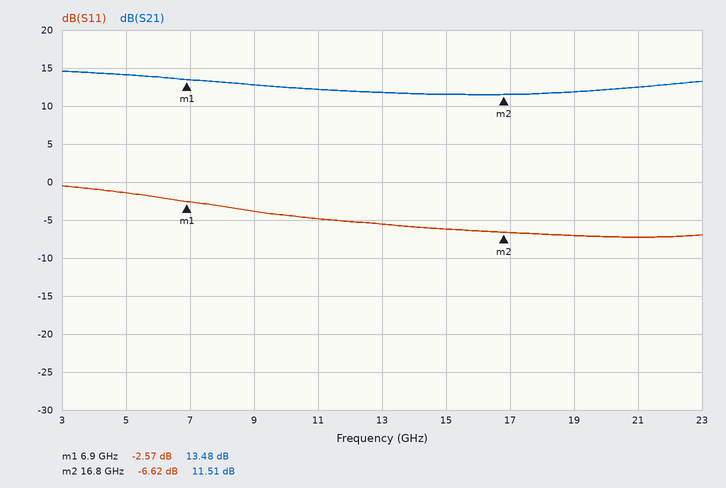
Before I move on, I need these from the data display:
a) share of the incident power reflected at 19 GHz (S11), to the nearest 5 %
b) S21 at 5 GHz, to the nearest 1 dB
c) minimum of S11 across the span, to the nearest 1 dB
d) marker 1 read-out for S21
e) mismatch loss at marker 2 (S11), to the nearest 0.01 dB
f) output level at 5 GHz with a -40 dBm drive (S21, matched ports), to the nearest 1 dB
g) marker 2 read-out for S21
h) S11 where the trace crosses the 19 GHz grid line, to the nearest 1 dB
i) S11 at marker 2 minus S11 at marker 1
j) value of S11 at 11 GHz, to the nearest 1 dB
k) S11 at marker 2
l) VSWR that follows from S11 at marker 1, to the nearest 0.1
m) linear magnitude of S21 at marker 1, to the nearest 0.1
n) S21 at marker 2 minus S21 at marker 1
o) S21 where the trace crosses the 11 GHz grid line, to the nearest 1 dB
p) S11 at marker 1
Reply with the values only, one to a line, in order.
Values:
20 %
14 dB
-7 dB
13.48 dB
1.07 dB
-26 dBm
11.51 dB
-7 dB
-4.05 dB
-5 dB
-6.62 dB
6.8
4.7
-1.97 dB
12 dB
-2.57 dB
